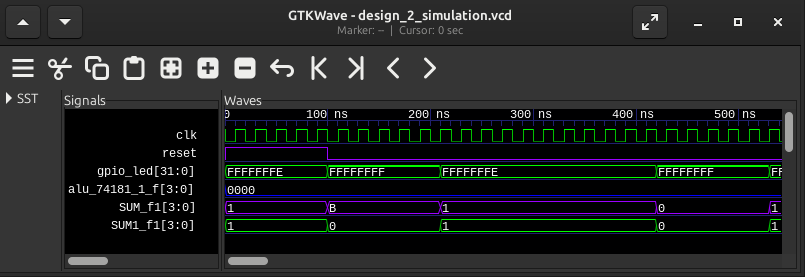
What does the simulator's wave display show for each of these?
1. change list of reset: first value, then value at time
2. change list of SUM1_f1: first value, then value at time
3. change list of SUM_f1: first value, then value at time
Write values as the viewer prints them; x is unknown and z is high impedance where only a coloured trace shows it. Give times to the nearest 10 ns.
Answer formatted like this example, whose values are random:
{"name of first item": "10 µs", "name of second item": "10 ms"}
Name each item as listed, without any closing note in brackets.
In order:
{"change list of reset: first value, then value at time": "1, 0 at 100 ns", "change list of SUM1_f1: first value, then value at time": "1, 0 at 100 ns, 1 at 210 ns, 0 at 420 ns, 1 at 530 ns", "change list of SUM_f1: first value, then value at time": "1, B at 100 ns, 1 at 210 ns, 0 at 420 ns, 1 at 530 ns"}
